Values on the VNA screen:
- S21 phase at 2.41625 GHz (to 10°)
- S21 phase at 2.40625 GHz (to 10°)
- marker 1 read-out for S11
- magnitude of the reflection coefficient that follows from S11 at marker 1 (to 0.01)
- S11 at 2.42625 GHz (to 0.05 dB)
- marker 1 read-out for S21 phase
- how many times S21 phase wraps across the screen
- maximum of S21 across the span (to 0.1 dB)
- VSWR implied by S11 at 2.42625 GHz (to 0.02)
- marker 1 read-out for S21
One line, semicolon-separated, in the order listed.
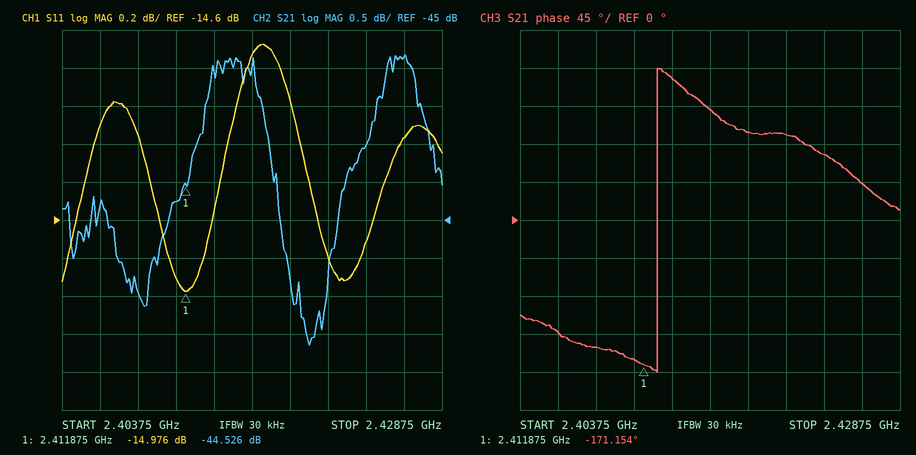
130°; -130°; -14.976 dB; 0.18; -14.15 dB; -171.154°; 1; -42.8 dB; 1.48; -44.526 dB
